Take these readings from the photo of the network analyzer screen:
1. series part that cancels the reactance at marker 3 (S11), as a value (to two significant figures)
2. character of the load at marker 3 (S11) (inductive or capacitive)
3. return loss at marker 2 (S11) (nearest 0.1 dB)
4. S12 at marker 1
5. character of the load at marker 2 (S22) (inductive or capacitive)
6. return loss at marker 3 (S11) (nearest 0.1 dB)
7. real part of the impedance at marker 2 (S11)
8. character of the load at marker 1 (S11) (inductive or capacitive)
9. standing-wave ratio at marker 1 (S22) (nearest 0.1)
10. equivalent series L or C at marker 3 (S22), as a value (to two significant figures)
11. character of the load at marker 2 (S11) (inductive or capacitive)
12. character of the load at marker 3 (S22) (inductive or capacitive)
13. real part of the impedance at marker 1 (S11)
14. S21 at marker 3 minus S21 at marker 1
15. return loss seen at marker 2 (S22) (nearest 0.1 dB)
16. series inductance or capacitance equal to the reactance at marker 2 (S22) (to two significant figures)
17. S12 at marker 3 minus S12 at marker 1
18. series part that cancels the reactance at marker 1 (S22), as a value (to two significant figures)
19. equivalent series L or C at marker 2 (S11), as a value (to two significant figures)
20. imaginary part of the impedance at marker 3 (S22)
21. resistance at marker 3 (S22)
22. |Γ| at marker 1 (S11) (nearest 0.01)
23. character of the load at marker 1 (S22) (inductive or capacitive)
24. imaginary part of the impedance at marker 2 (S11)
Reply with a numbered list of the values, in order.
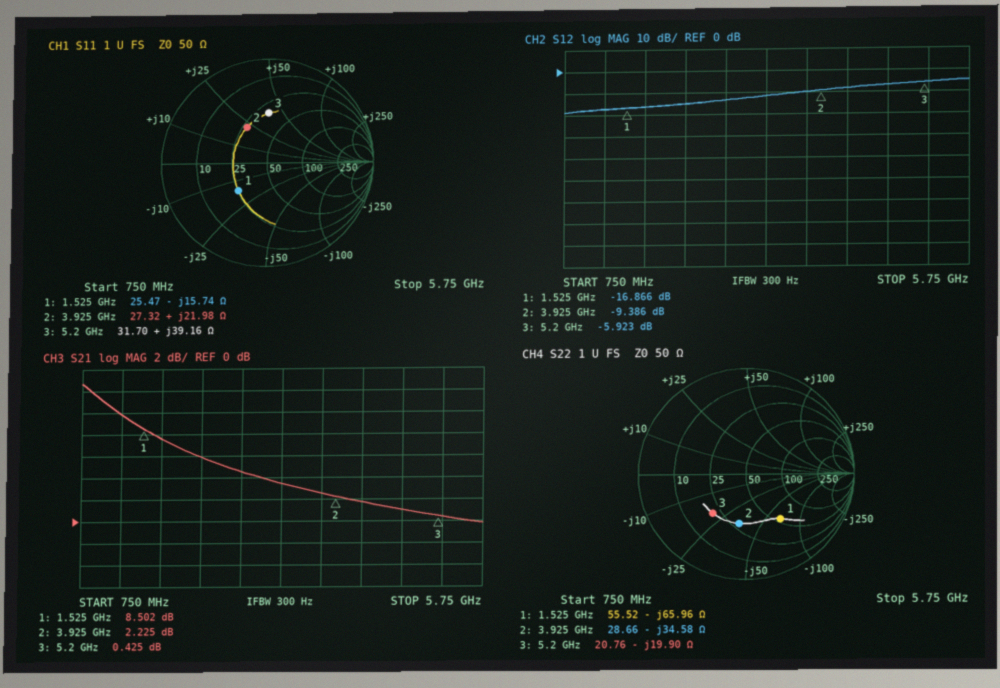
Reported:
1. 780 fF
2. inductive
3. 8.1 dB
4. -16.866 dB
5. capacitive
6. 6.4 dB
7. 27.32 Ω
8. capacitive
9. 3.3
10. 1.5 pF
11. inductive
12. capacitive
13. 25.47 Ω
14. -8.077 dB
15. 6.5 dB
16. 1.2 pF
17. 10.943 dB
18. 6.9 nH
19. 890 pH
20. -19.90 Ω
21. 20.76 Ω
22. 0.38
23. capacitive
24. +21.98 Ω
